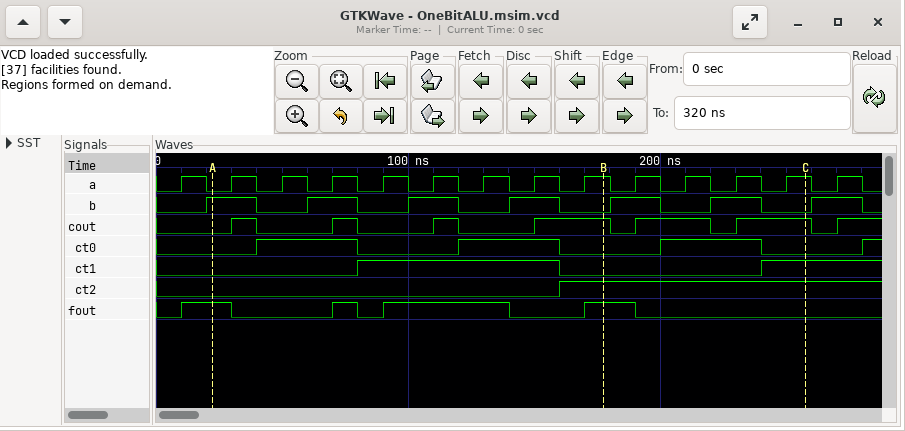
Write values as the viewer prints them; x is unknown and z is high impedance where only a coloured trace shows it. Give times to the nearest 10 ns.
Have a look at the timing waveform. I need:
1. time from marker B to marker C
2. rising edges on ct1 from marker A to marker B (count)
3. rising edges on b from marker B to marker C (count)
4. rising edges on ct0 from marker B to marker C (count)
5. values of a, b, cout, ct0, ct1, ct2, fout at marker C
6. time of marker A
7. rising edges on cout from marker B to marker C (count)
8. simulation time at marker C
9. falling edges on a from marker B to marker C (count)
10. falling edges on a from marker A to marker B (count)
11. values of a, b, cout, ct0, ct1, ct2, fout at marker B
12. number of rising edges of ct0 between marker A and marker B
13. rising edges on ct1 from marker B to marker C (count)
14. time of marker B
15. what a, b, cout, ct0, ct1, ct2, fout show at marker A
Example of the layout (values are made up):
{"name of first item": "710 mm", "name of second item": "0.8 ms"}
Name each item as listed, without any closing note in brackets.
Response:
{"time from marker B to marker C": "80 ns", "rising edges on ct1 from marker A to marker B": "1", "rising edges on b from marker B to marker C": "2", "rising edges on ct0 from marker B to marker C": "1", "values of a, b, cout, ct0, ct1, ct2, fout at marker C": "a=1, b=0, cout=1, ct0=0, ct1=1, ct2=1, fout=0", "time of marker A": "20 ns", "rising edges on cout from marker B to marker C": "2", "simulation time at marker C": "260 ns", "falling edges on a from marker B to marker C": "4", "falling edges on a from marker A to marker B": "7", "values of a, b, cout, ct0, ct1, ct2, fout at marker B": "a=1, b=0, cout=1, ct0=0, ct1=0, ct2=1, fout=1", "number of rising edges of ct0 between marker A and marker B": "2", "rising edges on ct1 from marker B to marker C": "1", "time of marker B": "180 ns", "what a, b, cout, ct0, ct1, ct2, fout show at marker A": "a=0, b=1, cout=0, ct0=0, ct1=0, ct2=0, fout=1"}
